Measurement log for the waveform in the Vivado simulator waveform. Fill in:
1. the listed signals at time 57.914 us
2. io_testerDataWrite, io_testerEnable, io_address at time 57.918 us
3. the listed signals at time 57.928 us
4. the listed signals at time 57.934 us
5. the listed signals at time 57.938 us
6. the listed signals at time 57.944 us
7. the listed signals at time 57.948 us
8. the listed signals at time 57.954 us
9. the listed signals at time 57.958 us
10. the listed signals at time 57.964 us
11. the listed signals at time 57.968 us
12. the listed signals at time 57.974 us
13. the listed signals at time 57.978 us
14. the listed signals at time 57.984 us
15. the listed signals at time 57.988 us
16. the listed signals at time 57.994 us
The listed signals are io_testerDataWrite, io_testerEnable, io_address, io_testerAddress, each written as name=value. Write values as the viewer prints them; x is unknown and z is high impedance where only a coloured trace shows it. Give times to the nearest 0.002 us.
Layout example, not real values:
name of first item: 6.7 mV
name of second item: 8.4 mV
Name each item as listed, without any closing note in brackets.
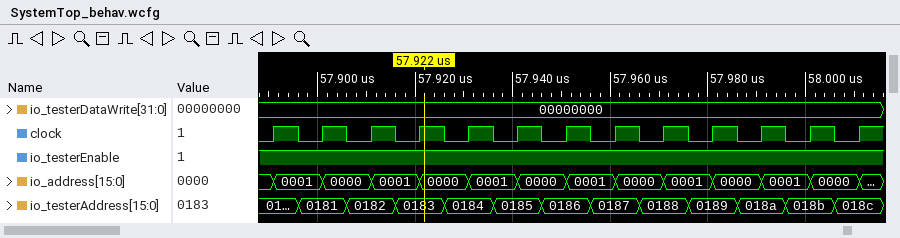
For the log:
the listed signals at time 57.914 us: io_testerDataWrite=00000000, io_testerEnable=1, io_address=0001, io_testerAddress=0182
io_testerDataWrite, io_testerEnable, io_address at time 57.918 us: io_testerDataWrite=00000000, io_testerEnable=1, io_address=0001
the listed signals at time 57.928 us: io_testerDataWrite=00000000, io_testerEnable=1, io_address=0000, io_testerAddress=0184
the listed signals at time 57.934 us: io_testerDataWrite=00000000, io_testerEnable=1, io_address=0001, io_testerAddress=0184
the listed signals at time 57.938 us: io_testerDataWrite=00000000, io_testerEnable=1, io_address=0001, io_testerAddress=0185
the listed signals at time 57.944 us: io_testerDataWrite=00000000, io_testerEnable=1, io_address=0000, io_testerAddress=0185
the listed signals at time 57.948 us: io_testerDataWrite=00000000, io_testerEnable=1, io_address=0000, io_testerAddress=0186
the listed signals at time 57.954 us: io_testerDataWrite=00000000, io_testerEnable=1, io_address=0001, io_testerAddress=0186
the listed signals at time 57.958 us: io_testerDataWrite=00000000, io_testerEnable=1, io_address=0001, io_testerAddress=0187
the listed signals at time 57.964 us: io_testerDataWrite=00000000, io_testerEnable=1, io_address=0000, io_testerAddress=0187
the listed signals at time 57.968 us: io_testerDataWrite=00000000, io_testerEnable=1, io_address=0000, io_testerAddress=0188
the listed signals at time 57.974 us: io_testerDataWrite=00000000, io_testerEnable=1, io_address=0001, io_testerAddress=0188
the listed signals at time 57.978 us: io_testerDataWrite=00000000, io_testerEnable=1, io_address=0001, io_testerAddress=0189
the listed signals at time 57.984 us: io_testerDataWrite=00000000, io_testerEnable=1, io_address=0000, io_testerAddress=0189
the listed signals at time 57.988 us: io_testerDataWrite=00000000, io_testerEnable=1, io_address=0000, io_testerAddress=018a
the listed signals at time 57.994 us: io_testerDataWrite=00000000, io_testerEnable=1, io_address=0001, io_testerAddress=018a
